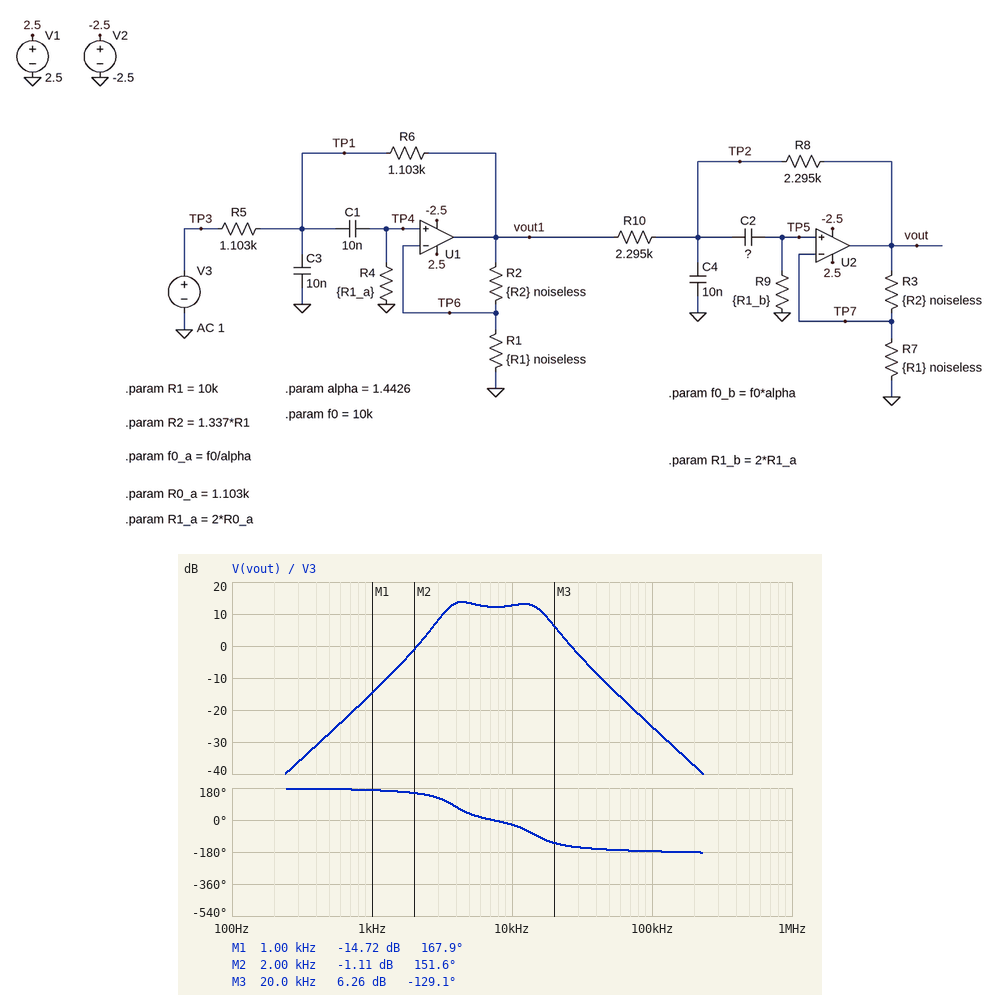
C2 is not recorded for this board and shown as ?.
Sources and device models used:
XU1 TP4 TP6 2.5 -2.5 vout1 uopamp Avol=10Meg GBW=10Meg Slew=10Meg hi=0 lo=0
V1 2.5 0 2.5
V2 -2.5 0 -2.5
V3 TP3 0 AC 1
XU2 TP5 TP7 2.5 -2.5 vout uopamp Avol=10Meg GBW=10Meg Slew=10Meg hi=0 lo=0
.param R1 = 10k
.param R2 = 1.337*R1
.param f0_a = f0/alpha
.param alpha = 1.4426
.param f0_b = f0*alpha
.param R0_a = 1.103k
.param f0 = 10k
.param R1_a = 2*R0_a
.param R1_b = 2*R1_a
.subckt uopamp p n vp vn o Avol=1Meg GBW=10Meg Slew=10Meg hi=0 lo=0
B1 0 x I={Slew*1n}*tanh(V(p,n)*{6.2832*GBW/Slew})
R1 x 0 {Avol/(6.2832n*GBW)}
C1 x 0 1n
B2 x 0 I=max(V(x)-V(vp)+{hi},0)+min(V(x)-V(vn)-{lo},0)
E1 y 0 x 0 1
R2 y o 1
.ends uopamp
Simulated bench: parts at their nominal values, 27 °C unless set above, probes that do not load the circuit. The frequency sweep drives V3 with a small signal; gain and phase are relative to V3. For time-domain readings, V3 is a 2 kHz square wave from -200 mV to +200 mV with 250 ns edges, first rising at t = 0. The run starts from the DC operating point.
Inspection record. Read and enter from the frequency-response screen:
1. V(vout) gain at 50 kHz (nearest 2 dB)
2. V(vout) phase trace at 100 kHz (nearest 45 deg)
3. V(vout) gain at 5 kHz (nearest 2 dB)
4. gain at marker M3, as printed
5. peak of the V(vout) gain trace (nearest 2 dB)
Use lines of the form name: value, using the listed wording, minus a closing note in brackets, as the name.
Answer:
V(vout) gain at 50 kHz: -12 dB
V(vout) phase trace at 100 kHz: -180 deg
V(vout) gain at 5 kHz: 14 dB
gain at marker M3, as printed: 6.26 dB
peak of the V(vout) gain trace: 14 dB
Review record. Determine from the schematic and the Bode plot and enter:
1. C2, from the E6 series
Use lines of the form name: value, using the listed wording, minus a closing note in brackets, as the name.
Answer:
C2, from the E6 series: 33 nF
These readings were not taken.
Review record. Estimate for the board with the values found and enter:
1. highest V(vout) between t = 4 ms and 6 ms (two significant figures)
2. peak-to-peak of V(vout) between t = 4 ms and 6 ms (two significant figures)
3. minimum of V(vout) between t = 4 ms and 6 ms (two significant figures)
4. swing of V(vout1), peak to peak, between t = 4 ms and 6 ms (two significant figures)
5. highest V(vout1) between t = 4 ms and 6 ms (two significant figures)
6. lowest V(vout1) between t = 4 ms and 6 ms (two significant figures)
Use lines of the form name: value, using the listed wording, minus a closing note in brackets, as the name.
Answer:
highest V(vout) between t = 4 ms and 6 ms: 870 mV
peak-to-peak of V(vout) between t = 4 ms and 6 ms: 1.7 V
minimum of V(vout) between t = 4 ms and 6 ms: -870 mV
swing of V(vout1), peak to peak, between t = 4 ms and 6 ms: 1.2 V
highest V(vout1) between t = 4 ms and 6 ms: 610 mV
lowest V(vout1) between t = 4 ms and 6 ms: -610 mV
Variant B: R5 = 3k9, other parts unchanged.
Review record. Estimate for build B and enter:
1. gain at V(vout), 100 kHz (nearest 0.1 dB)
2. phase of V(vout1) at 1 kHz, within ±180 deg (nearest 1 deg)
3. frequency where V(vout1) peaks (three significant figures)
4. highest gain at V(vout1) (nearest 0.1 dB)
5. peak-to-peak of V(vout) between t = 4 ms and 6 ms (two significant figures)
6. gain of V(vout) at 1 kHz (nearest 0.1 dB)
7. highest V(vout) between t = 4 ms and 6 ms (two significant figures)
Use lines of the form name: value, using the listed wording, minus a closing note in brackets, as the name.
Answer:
gain at V(vout), 100 kHz: -36.2 dB
phase of V(vout1) at 1 kHz, within ±180 deg: 90 deg
frequency where V(vout1) peaks: 11.5 kHz
highest gain at V(vout1): 21.7 dB
peak-to-peak of V(vout) between t = 4 ms and 6 ms: 5.0 V
gain of V(vout) at 1 kHz: -21.8 dB
highest V(vout) between t = 4 ms and 6 ms: 2.5 V
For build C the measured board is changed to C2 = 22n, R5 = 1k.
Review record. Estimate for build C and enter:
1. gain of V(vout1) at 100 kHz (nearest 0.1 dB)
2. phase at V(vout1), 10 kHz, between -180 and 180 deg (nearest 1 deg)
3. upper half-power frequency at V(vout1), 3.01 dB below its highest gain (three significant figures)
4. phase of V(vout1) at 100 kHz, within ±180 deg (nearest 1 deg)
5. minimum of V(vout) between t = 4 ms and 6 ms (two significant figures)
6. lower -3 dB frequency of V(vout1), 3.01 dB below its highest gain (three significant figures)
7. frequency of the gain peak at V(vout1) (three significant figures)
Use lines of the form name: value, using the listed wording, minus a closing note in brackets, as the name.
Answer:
gain of V(vout1) at 100 kHz: -8.5 dB
phase at V(vout1), 10 kHz, between -180 and 180 deg: 47 deg
upper half-power frequency at V(vout1), 3.01 dB below its highest gain: 21.2 kHz
phase of V(vout1) at 100 kHz, within ±180 deg: -85 deg
minimum of V(vout) between t = 4 ms and 6 ms: -940 mV
lower -3 dB frequency of V(vout1), 3.01 dB below its highest gain: 10.2 kHz
frequency of the gain peak at V(vout1): 14.7 kHz
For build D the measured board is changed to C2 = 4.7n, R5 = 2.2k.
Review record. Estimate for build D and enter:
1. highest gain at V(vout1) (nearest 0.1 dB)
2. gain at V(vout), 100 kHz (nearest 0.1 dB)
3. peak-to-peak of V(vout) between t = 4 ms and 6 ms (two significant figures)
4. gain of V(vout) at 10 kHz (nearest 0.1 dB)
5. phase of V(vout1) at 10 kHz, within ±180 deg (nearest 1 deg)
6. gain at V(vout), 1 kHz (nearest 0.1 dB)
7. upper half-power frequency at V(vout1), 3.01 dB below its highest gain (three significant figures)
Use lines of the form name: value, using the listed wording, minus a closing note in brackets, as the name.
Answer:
highest gain at V(vout1): 17.1 dB
gain at V(vout), 100 kHz: -31.2 dB
peak-to-peak of V(vout) between t = 4 ms and 6 ms: 1.1 V
gain of V(vout) at 10 kHz: 14.1 dB
phase of V(vout1) at 10 kHz, within ±180 deg: 67 deg
gain at V(vout), 1 kHz: -35.6 dB
upper half-power frequency at V(vout1), 3.01 dB below its highest gain: 13.7 kHz
